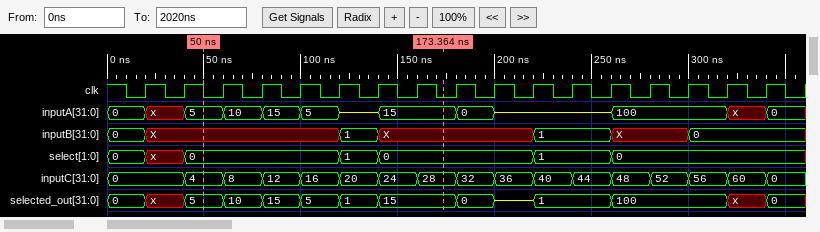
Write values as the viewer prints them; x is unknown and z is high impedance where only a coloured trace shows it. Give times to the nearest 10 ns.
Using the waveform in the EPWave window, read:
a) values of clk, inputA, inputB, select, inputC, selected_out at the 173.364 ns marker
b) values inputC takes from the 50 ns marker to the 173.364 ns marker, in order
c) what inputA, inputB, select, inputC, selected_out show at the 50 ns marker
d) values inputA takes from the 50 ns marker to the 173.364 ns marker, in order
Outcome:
clk=0, inputA=15, inputB=X, select=0, inputC=28, selected_out=15
4, 8, 12, 16, 20, 24, 28
inputA=5, inputB=X, select=0, inputC=4, selected_out=5
5, 10, 15, 5, z, 15
